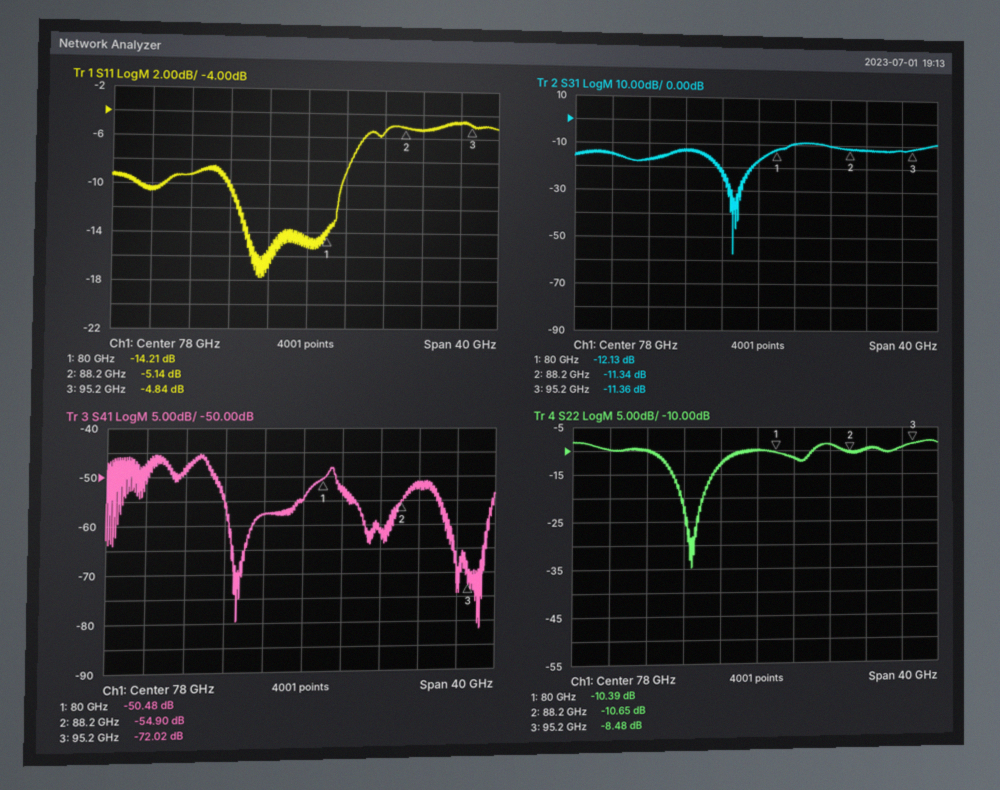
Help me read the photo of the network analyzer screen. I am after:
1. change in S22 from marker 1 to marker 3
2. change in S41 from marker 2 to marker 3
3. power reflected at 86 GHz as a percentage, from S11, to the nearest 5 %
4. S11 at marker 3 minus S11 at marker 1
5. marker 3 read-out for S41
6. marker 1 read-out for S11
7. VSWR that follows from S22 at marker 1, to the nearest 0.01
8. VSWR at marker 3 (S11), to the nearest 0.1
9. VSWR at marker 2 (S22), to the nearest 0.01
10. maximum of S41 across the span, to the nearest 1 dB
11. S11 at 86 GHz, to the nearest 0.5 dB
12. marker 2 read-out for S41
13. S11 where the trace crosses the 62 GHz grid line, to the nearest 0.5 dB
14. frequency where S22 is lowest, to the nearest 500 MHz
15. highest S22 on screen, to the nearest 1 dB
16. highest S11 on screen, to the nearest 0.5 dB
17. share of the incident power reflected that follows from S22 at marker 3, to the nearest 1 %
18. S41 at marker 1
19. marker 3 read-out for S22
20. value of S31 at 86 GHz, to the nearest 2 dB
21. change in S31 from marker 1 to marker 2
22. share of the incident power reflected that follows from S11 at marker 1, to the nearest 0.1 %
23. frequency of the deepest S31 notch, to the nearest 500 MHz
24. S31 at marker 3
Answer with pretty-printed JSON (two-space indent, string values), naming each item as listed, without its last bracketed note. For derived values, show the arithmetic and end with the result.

{
  "change in S22 from marker 1 to marker 3": "-8.48 − (-10.39) = 1.91 dB",
  "change in S41 from marker 2 to marker 3": "-72.02 − (-54.9) = -17.12 dB",
  "power reflected at 86 GHz as a percentage, from S11, to the nearest 5 %": "10^(-5.5/10) ≈ 28.2 %, so 30 % to the nearest 5 %",
  "S11 at marker 3 minus S11 at marker 1": "-4.84 − (-14.21) = 9.37 dB",
  "marker 3 read-out for S41": "-72.02 dB",
  "marker 1 read-out for S11": "-14.21 dB",
  "VSWR that follows from S22 at marker 1, to the nearest 0.01": "(1 + 0.3023)/(1 − 0.3023) ≈ 1.87",
  "VSWR at marker 3 (S11), to the nearest 0.1": "(1 + 0.5728)/(1 − 0.5728) ≈ 3.7",
  "VSWR at marker 2 (S22), to the nearest 0.01": "(1 + 0.2934)/(1 − 0.2934) ≈ 1.83",
  "maximum of S41 across the span, to the nearest 1 dB": "-45 dB",
  "S11 at 86 GHz, to the nearest 0.5 dB": "-5.5 dB",
  "marker 2 read-out for S41": "-54.90 dB",
  "S11 where the trace crosses the 62 GHz grid line, to the nearest 0.5 dB": "-10.5 dB",
  "frequency where S22 is lowest, to the nearest 500 MHz": "71.0 GHz",
  "highest S22 on screen, to the nearest 1 dB": "-8 dB",
  "highest S11 on screen, to the nearest 0.5 dB": "-4.5 dB",
  "share of the incident power reflected that follows from S22 at marker 3, to the nearest 1 %": "10^(-8.48/10) ≈ 14 %",
  "S41 at marker 1": "-50.48 dB",
  "marker 3 read-out for S22": "-8.48 dB",
  "value of S31 at 86 GHz, to the nearest 2 dB": "-10 dB",
  "change in S31 from marker 1 to marker 2": "-11.34 − (-12.13) = 0.79 dB",
  "share of the incident power reflected that follows from S11 at marker 1, to the nearest 0.1 %": "10^(-14.21/10) ≈ 3.8 %",
  "frequency of the deepest S31 notch, to the nearest 500 MHz": "75.0 GHz",
  "S31 at marker 3": "-11.36 dB"
}
